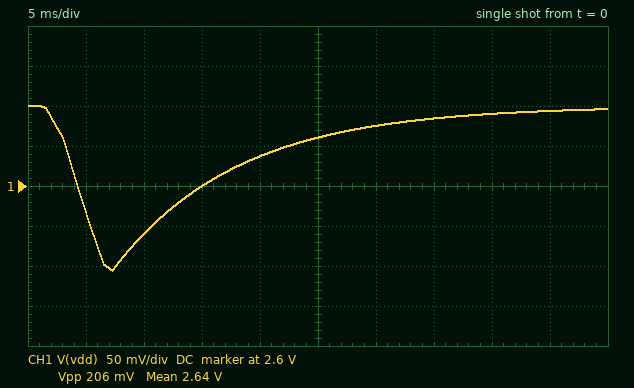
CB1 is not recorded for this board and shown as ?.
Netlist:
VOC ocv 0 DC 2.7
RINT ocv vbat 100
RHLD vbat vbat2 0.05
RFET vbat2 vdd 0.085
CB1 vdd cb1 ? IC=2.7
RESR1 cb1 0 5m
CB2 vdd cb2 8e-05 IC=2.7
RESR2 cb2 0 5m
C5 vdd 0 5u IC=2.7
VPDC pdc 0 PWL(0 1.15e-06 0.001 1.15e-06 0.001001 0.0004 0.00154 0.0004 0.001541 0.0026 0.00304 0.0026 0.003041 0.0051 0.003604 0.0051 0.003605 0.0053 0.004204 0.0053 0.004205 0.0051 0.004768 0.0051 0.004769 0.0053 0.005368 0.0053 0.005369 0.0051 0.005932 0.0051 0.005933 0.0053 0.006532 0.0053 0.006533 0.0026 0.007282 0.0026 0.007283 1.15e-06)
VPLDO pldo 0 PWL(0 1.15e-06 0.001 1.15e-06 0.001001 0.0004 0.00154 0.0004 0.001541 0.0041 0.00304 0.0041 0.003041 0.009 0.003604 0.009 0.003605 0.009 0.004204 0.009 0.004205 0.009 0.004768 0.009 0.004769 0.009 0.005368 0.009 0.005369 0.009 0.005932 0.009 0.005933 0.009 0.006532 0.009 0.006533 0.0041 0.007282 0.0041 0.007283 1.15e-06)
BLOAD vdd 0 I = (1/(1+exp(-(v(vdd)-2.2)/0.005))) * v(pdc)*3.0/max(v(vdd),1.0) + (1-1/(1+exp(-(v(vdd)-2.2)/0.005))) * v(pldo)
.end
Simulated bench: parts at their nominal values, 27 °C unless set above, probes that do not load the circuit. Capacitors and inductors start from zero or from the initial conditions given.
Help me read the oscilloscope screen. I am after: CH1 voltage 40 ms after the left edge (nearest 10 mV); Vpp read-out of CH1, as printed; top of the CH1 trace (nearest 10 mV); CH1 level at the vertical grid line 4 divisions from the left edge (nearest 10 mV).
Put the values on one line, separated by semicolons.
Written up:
2.69 V; 206 mV; 2.70 V; 2.64 V
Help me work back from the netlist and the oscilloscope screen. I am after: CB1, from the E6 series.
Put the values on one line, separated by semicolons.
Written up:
22 µF
